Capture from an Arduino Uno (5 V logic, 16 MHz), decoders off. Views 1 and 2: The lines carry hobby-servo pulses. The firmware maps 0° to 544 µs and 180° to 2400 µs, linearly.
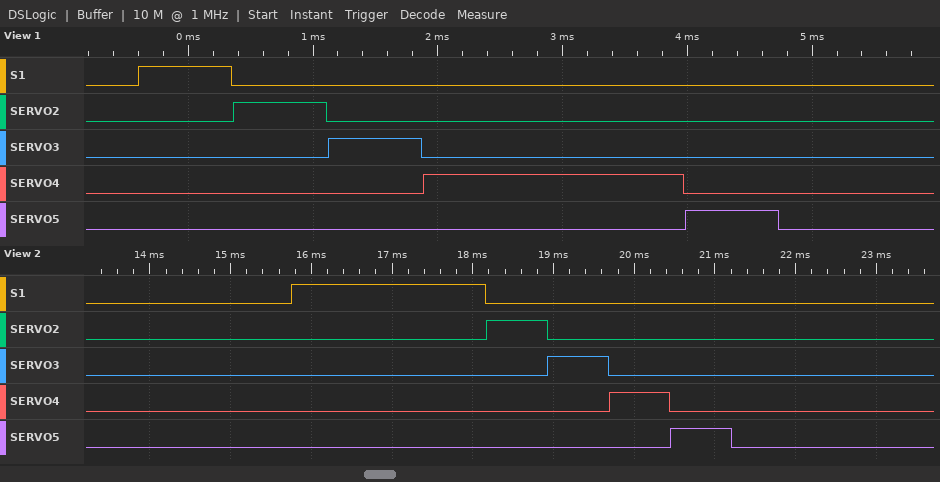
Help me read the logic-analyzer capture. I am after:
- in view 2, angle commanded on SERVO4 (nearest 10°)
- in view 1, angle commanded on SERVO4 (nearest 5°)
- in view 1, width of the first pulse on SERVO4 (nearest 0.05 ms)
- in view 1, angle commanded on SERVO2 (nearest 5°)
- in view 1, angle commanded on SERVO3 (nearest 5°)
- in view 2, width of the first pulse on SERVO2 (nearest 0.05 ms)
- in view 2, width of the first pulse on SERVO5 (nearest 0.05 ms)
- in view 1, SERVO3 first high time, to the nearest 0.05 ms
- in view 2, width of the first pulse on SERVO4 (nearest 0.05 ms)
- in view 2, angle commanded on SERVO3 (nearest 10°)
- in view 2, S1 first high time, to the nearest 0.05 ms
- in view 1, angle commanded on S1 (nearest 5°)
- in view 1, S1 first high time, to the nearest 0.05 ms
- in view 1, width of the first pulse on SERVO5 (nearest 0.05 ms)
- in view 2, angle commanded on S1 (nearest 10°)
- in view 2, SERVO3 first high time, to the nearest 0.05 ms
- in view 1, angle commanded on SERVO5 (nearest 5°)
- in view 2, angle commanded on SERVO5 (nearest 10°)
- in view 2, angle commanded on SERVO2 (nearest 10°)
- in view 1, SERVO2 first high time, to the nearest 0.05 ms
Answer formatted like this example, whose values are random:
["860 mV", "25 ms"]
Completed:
["20°", "150°", "2.10 ms", "20°", "20°", "0.75 ms", "0.75 ms", "0.75 ms", "0.75 ms", "20°", "2.40 ms", "20°", "0.75 ms", "0.75 ms", "180°", "0.75 ms", "20°", "20°", "20°", "0.75 ms"]
